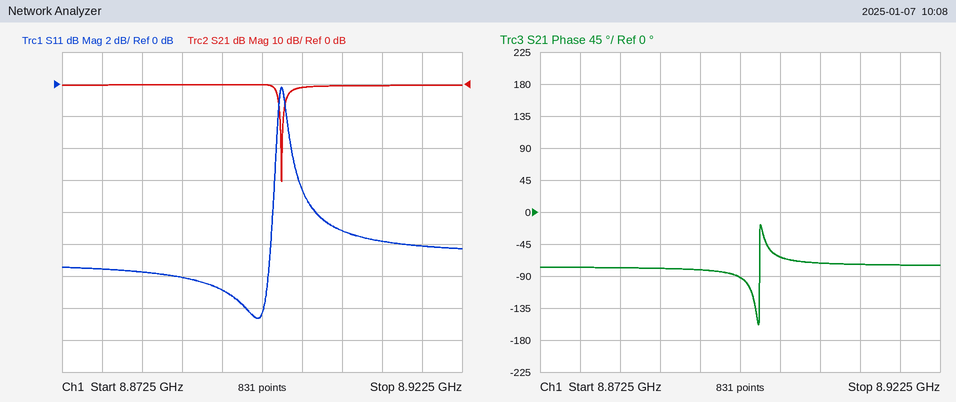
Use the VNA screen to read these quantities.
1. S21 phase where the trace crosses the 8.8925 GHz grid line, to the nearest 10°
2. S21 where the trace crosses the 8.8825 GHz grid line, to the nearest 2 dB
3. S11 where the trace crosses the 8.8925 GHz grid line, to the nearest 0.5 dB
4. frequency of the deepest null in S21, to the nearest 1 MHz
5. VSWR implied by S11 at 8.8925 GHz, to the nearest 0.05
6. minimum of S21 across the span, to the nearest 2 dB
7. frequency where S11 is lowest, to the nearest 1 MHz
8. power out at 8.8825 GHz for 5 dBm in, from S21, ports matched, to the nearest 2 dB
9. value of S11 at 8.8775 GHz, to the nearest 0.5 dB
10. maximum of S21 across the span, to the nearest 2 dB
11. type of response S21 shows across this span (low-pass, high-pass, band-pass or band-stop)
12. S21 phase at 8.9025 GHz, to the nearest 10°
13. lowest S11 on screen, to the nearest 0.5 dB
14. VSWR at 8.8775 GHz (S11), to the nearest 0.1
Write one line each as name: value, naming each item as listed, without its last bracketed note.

S21 phase where the trace crosses the 8.8925 GHz grid line, to the nearest 10°: -80°
S21 where the trace crosses the 8.8825 GHz grid line, to the nearest 2 dB: 0 dB
S11 where the trace crosses the 8.8925 GHz grid line, to the nearest 0.5 dB: -13.0 dB
frequency of the deepest null in S21, to the nearest 1 MHz: 8.900 GHz
VSWR implied by S11 at 8.8925 GHz, to the nearest 0.05: 1.60
minimum of S21 across the span, to the nearest 2 dB: -30 dB
frequency where S11 is lowest, to the nearest 1 MHz: 8.897 GHz
power out at 8.8825 GHz for 5 dBm in, from S21, ports matched, to the nearest 2 dB: 4 dBm
value of S11 at 8.8775 GHz, to the nearest 0.5 dB: -11.5 dB
maximum of S21 across the span, to the nearest 2 dB: 0 dB
type of response S21 shows across this span: band-stop
S21 phase at 8.9025 GHz, to the nearest 10°: -60°
lowest S11 on screen, to the nearest 0.5 dB: -14.5 dB
VSWR at 8.8775 GHz (S11), to the nearest 0.1: 1.7
